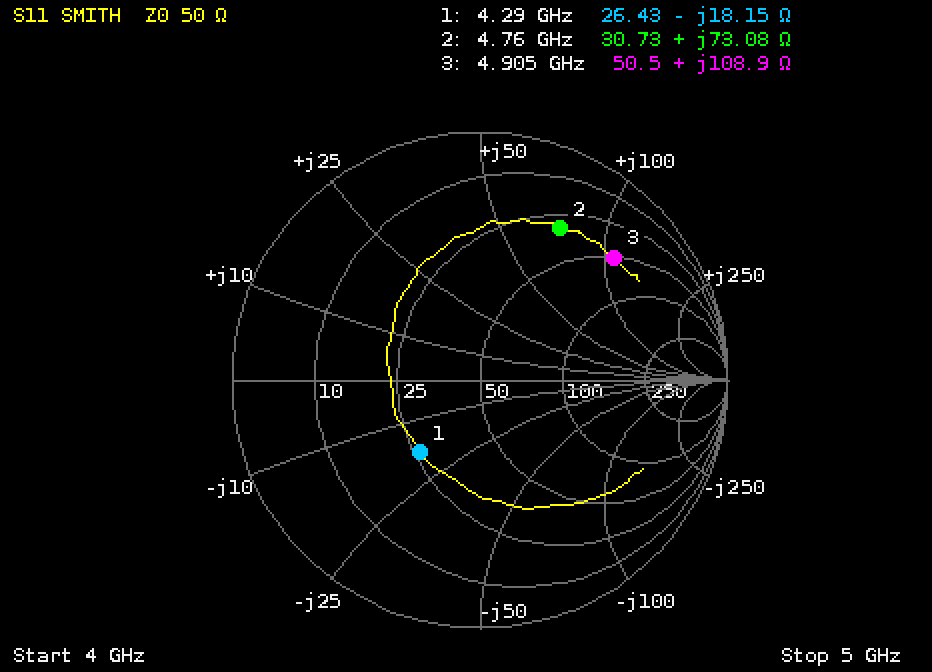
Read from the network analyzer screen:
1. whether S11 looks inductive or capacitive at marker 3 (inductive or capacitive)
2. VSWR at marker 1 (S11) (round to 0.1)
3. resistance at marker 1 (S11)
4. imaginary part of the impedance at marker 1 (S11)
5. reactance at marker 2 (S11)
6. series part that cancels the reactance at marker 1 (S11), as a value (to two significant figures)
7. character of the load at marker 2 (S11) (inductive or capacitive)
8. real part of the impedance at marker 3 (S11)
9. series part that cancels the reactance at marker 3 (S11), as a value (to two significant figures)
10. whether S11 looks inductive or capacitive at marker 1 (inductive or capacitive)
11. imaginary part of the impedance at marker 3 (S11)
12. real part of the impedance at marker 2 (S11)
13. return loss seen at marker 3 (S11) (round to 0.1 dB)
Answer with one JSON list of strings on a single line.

["inductive", "2.2", "26.43 Ω", "-18.15 Ω", "+73.08 Ω", "670 pH", "inductive", "50.5 Ω", "300 fF", "capacitive", "+108.9 Ω", "30.73 Ω", "2.7 dB"]
